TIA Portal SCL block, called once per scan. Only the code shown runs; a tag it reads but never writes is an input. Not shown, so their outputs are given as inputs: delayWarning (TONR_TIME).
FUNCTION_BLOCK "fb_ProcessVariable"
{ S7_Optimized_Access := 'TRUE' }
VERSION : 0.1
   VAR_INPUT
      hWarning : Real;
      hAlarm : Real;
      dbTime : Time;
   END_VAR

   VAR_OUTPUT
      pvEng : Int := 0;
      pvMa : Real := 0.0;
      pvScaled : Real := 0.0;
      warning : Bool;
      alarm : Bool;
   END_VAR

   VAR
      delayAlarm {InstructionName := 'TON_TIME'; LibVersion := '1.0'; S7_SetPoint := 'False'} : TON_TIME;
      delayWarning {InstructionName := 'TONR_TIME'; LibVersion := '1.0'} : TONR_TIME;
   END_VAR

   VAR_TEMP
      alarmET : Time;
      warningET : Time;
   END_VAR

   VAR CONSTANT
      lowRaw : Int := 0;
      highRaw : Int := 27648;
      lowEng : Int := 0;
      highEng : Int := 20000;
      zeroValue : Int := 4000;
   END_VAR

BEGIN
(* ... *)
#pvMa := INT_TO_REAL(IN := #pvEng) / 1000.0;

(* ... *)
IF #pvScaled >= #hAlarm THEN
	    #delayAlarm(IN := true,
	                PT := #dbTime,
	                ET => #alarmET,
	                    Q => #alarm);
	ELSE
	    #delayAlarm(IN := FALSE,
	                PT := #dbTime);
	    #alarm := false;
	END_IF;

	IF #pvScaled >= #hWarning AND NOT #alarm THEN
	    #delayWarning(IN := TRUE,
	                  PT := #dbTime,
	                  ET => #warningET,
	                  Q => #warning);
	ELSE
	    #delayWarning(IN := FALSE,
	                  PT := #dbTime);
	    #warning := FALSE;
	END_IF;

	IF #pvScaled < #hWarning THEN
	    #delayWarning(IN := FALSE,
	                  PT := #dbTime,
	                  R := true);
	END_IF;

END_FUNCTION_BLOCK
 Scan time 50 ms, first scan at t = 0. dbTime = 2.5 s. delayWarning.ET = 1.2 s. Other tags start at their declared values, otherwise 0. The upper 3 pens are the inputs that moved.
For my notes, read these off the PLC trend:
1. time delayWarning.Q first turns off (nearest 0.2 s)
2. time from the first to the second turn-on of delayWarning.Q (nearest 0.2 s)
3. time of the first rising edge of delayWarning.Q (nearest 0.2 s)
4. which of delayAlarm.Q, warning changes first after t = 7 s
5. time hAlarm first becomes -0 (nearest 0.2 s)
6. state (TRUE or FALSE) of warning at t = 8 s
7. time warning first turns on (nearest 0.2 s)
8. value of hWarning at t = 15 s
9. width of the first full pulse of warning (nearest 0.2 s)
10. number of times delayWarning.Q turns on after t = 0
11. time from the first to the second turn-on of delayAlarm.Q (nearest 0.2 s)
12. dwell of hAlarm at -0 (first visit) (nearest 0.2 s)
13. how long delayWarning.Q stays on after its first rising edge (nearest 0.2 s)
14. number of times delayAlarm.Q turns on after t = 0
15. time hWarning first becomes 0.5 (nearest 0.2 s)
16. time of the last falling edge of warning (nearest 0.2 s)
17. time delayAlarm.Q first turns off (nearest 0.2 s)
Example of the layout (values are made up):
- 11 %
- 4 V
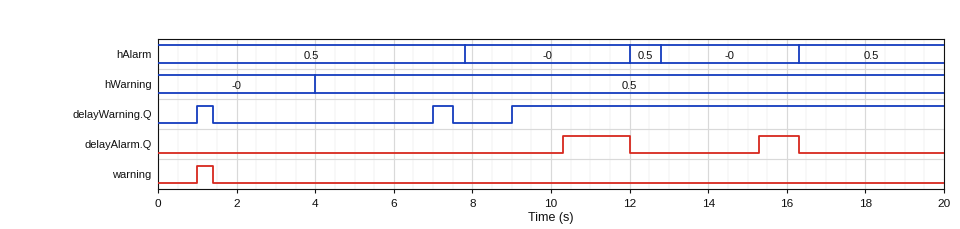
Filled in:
- 1.4 s
- 6.0 s
- 1.0 s
- delayAlarm.Q
- 7.8 s
- FALSE
- 1.0 s
- 0.5
- 0.4 s
- 3
- 5.0 s
- 4.2 s
- 0.4 s
- 2
- 4.0 s
- 1.4 s
- 12.0 s
